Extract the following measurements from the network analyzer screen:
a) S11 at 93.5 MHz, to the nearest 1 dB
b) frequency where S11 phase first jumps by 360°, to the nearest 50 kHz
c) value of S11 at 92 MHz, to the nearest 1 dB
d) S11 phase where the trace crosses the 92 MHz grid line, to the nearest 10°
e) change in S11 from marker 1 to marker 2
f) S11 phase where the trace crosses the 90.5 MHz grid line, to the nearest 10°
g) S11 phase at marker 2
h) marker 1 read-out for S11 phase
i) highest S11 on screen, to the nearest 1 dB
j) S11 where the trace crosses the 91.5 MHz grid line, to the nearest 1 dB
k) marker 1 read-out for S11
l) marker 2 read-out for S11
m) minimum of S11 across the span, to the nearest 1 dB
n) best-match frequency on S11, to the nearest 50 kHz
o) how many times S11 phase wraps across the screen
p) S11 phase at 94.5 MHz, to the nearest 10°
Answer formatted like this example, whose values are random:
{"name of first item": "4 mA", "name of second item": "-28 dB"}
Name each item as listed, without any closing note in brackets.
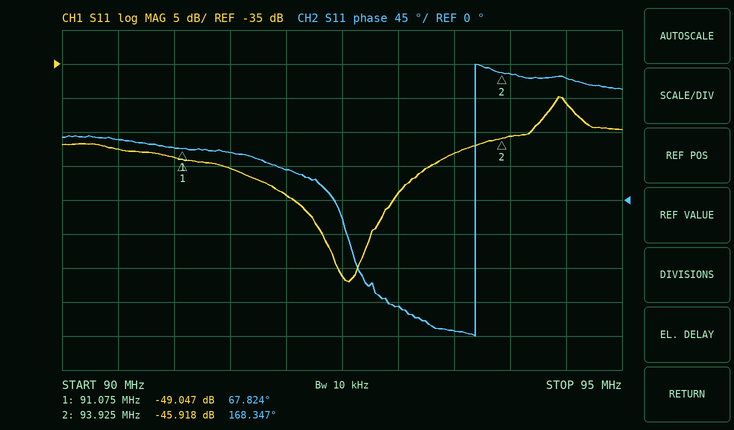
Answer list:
{"S11 at 93.5 MHz, to the nearest 1 dB": "-48 dB", "frequency where S11 phase first jumps by 360°, to the nearest 50 kHz": "93.70 MHz", "value of S11 at 92 MHz, to the nearest 1 dB": "-54 dB", "S11 phase where the trace crosses the 92 MHz grid line, to the nearest 10°": "40°", "change in S11 from marker 1 to marker 2": "3.129 dB", "S11 phase where the trace crosses the 90.5 MHz grid line, to the nearest 10°": "80°", "S11 phase at marker 2": "168.347°", "marker 1 read-out for S11 phase": "67.824°", "highest S11 on screen, to the nearest 1 dB": "-40 dB", "S11 where the trace crosses the 91.5 MHz grid line, to the nearest 1 dB": "-50 dB", "marker 1 read-out for S11": "-49.047 dB", "marker 2 read-out for S11": "-45.918 dB", "minimum of S11 across the span, to the nearest 1 dB": "-67 dB", "best-match frequency on S11, to the nearest 50 kHz": "92.55 MHz", "how many times S11 phase wraps across the screen": "1", "S11 phase at 94.5 MHz, to the nearest 10°": "160°"}
